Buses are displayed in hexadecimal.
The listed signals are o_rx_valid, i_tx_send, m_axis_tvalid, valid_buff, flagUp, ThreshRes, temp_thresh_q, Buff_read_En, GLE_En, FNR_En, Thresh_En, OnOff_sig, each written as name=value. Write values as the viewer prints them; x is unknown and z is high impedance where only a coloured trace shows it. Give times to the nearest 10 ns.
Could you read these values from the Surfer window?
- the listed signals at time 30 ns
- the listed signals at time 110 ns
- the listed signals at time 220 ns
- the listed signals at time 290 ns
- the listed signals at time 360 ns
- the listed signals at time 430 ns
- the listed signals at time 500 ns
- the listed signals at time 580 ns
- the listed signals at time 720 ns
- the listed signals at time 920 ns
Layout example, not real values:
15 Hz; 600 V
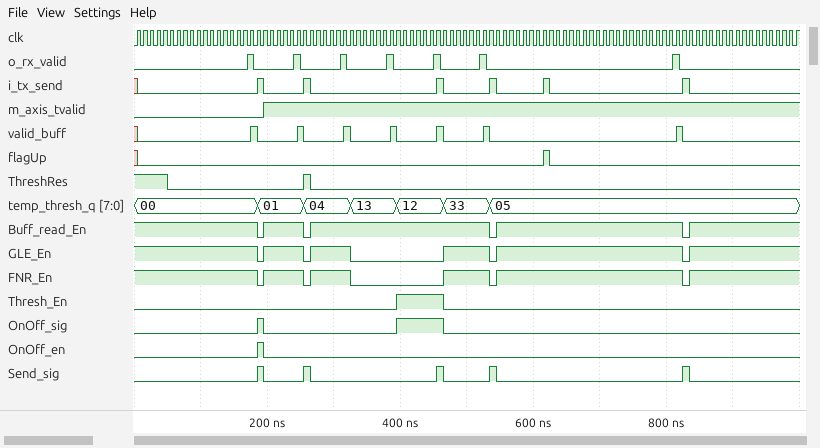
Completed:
o_rx_valid=0, i_tx_send=0, m_axis_tvalid=0, valid_buff=0, flagUp=0, ThreshRes=1, temp_thresh_q=00, Buff_read_En=1, GLE_En=1, FNR_En=1, Thresh_En=0, OnOff_sig=0; o_rx_valid=0, i_tx_send=0, m_axis_tvalid=0, valid_buff=0, flagUp=0, ThreshRes=0, temp_thresh_q=00, Buff_read_En=1, GLE_En=1, FNR_En=1, Thresh_En=0, OnOff_sig=0; o_rx_valid=0, i_tx_send=0, m_axis_tvalid=1, valid_buff=0, flagUp=0, ThreshRes=0, temp_thresh_q=01, Buff_read_En=1, GLE_En=1, FNR_En=1, Thresh_En=0, OnOff_sig=0; o_rx_valid=0, i_tx_send=0, m_axis_tvalid=1, valid_buff=0, flagUp=0, ThreshRes=0, temp_thresh_q=04, Buff_read_En=1, GLE_En=1, FNR_En=1, Thresh_En=0, OnOff_sig=0; o_rx_valid=0, i_tx_send=0, m_axis_tvalid=1, valid_buff=0, flagUp=0, ThreshRes=0, temp_thresh_q=13, Buff_read_En=1, GLE_En=0, FNR_En=0, Thresh_En=0, OnOff_sig=0; o_rx_valid=0, i_tx_send=0, m_axis_tvalid=1, valid_buff=0, flagUp=0, ThreshRes=0, temp_thresh_q=12, Buff_read_En=1, GLE_En=0, FNR_En=0, Thresh_En=1, OnOff_sig=1; o_rx_valid=0, i_tx_send=0, m_axis_tvalid=1, valid_buff=0, flagUp=0, ThreshRes=0, temp_thresh_q=33, Buff_read_En=1, GLE_En=1, FNR_En=1, Thresh_En=0, OnOff_sig=0; o_rx_valid=0, i_tx_send=0, m_axis_tvalid=1, valid_buff=0, flagUp=0, ThreshRes=0, temp_thresh_q=05, Buff_read_En=1, GLE_En=1, FNR_En=1, Thresh_En=0, OnOff_sig=0; o_rx_valid=0, i_tx_send=0, m_axis_tvalid=1, valid_buff=0, flagUp=0, ThreshRes=0, temp_thresh_q=05, Buff_read_En=1, GLE_En=1, FNR_En=1, Thresh_En=0, OnOff_sig=0; o_rx_valid=0, i_tx_send=0, m_axis_tvalid=1, valid_buff=0, flagUp=0, ThreshRes=0, temp_thresh_q=05, Buff_read_En=1, GLE_En=1, FNR_En=1, Thresh_En=0, OnOff_sig=0
